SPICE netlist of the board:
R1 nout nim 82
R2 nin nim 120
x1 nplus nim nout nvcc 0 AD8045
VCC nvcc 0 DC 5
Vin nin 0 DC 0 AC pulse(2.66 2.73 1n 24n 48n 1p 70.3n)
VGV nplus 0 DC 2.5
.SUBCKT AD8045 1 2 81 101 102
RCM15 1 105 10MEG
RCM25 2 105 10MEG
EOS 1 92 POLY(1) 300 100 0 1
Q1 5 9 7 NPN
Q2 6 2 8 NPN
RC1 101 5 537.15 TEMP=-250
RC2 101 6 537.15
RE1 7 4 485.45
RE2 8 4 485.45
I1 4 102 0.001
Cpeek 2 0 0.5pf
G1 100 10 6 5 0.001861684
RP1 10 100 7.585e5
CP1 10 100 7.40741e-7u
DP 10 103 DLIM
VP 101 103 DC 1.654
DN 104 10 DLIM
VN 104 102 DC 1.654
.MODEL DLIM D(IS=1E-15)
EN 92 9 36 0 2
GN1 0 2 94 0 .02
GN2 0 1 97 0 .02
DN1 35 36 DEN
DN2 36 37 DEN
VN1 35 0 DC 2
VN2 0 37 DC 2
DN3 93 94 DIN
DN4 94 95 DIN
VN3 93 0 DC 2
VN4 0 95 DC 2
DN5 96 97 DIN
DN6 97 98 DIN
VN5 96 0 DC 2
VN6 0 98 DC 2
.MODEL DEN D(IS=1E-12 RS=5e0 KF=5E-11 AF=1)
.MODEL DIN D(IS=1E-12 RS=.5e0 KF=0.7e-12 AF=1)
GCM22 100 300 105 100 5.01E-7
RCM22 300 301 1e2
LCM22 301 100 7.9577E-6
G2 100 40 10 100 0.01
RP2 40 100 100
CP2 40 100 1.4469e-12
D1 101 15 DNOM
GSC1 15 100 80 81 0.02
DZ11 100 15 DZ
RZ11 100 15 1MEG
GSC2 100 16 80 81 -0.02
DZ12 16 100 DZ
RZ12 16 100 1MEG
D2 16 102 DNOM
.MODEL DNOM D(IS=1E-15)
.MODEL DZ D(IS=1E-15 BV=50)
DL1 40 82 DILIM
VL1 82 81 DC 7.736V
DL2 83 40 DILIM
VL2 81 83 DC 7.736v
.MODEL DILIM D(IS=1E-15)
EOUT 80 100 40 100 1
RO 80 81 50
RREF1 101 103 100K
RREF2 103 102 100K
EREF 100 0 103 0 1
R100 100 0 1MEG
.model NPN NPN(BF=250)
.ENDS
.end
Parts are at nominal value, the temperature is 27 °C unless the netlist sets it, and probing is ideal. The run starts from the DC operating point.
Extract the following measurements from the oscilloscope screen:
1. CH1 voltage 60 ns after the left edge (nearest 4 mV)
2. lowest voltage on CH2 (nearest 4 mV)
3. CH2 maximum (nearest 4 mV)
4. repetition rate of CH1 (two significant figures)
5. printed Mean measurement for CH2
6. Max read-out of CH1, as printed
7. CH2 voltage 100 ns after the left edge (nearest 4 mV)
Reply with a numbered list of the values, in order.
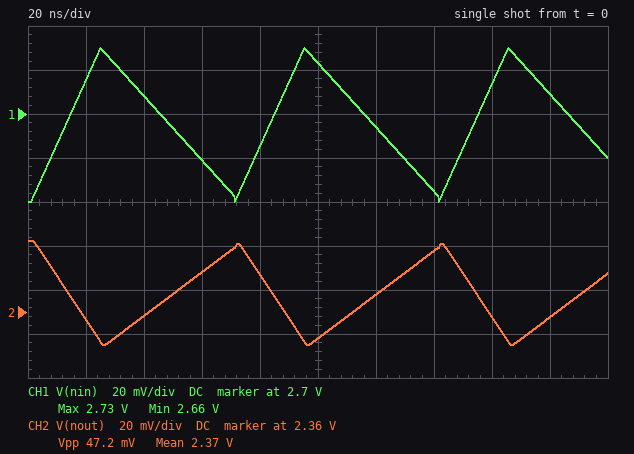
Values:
1. 2.680 V
2. 2.344 V
3. 2.392 V
4. 14 MHz
5. 2.37 V
6. 2.73 V
7. 2.348 V
